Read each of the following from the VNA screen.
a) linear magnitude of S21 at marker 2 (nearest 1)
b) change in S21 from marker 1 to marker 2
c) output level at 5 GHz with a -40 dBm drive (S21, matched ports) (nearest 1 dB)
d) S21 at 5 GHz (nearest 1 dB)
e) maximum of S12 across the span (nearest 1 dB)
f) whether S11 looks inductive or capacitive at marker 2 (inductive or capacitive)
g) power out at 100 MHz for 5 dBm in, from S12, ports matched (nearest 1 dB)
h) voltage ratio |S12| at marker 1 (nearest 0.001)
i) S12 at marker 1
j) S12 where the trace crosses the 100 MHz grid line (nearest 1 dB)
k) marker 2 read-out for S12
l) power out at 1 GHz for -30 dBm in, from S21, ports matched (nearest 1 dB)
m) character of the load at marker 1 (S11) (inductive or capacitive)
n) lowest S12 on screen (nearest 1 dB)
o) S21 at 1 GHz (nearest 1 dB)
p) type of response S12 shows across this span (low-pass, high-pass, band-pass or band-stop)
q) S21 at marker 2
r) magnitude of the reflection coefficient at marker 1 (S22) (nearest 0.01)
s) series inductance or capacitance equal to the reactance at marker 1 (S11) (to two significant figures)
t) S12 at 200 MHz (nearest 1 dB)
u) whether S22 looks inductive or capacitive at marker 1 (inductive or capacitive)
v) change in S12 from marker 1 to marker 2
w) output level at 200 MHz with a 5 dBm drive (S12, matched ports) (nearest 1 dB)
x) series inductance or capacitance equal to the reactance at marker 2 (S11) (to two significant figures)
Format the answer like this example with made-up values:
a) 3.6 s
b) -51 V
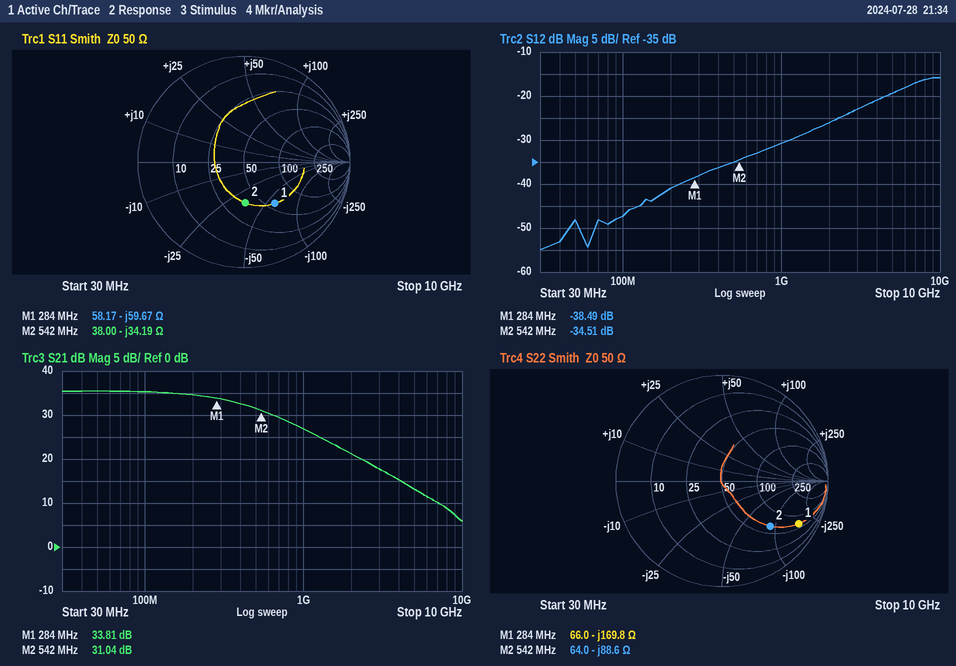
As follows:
a) 36
b) -2.77 dB
c) -27 dBm
d) 13 dB
e) -16 dB
f) capacitive
g) -42 dBm
h) 0.012
i) -38.49 dB
j) -47 dB
k) -34.51 dB
l) -3 dBm
m) capacitive
n) -55 dB
o) 27 dB
p) high-pass
q) 31.04 dB
r) 0.83
s) 9.4 pF
t) -41 dB
u) capacitive
v) 3.98 dB
w) -36 dBm
x) 8.6 pF
